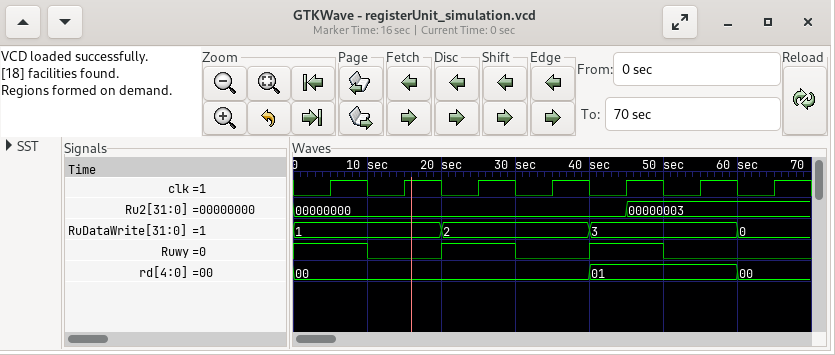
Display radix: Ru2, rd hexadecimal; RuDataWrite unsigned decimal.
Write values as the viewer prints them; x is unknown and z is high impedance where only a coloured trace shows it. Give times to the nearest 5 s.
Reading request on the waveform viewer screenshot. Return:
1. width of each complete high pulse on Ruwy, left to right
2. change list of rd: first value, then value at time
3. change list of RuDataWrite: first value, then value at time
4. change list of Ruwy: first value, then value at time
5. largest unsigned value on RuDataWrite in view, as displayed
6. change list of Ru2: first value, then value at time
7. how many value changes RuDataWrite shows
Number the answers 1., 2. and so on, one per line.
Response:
1. 10 s, 10 s
2. 00, 01 at 40 s, 00 at 60 s
3. 1, 2 at 20 s, 3 at 40 s, 0 at 60 s
4. 1, 0 at 10 s, 1 at 20 s, 0 at 30 s, 1 at 40 s, 0 at 50 s
5. 3
6. 00000000, 00000003 at 45 s
7. 3
